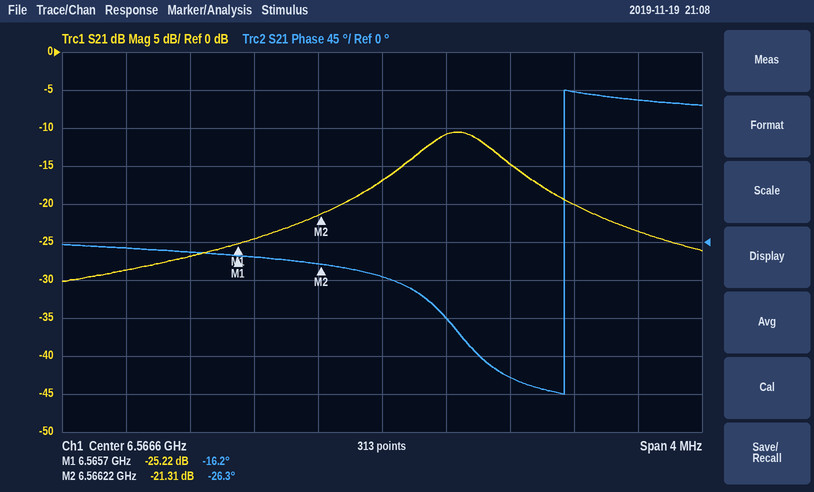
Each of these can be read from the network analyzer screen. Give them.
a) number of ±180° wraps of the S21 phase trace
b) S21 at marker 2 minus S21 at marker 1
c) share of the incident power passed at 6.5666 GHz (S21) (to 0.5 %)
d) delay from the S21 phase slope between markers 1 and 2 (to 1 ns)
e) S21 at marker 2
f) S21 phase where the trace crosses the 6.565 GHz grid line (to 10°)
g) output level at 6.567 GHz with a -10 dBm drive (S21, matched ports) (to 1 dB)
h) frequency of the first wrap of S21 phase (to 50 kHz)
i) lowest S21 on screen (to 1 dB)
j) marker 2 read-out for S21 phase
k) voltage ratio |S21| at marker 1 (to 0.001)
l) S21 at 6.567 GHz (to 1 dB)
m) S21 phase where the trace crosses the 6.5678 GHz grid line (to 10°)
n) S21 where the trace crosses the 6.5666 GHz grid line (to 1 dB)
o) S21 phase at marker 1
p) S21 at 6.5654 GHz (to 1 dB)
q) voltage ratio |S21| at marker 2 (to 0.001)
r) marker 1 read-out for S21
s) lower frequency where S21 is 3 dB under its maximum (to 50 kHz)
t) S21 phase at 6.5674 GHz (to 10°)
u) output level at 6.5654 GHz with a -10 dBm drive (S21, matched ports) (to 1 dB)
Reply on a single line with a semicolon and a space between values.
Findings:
1; 3.91 dB; 2.0 %; 54 ns; -21.31 dB; -10°; -21 dBm; 6.56775 GHz; -30 dB; -26.3°; 0.055; -11 dB; 180°; -17 dB; -16.2°; -27 dB; 0.086; -25.22 dB; 6.56680 GHz; -160°; -37 dBm
